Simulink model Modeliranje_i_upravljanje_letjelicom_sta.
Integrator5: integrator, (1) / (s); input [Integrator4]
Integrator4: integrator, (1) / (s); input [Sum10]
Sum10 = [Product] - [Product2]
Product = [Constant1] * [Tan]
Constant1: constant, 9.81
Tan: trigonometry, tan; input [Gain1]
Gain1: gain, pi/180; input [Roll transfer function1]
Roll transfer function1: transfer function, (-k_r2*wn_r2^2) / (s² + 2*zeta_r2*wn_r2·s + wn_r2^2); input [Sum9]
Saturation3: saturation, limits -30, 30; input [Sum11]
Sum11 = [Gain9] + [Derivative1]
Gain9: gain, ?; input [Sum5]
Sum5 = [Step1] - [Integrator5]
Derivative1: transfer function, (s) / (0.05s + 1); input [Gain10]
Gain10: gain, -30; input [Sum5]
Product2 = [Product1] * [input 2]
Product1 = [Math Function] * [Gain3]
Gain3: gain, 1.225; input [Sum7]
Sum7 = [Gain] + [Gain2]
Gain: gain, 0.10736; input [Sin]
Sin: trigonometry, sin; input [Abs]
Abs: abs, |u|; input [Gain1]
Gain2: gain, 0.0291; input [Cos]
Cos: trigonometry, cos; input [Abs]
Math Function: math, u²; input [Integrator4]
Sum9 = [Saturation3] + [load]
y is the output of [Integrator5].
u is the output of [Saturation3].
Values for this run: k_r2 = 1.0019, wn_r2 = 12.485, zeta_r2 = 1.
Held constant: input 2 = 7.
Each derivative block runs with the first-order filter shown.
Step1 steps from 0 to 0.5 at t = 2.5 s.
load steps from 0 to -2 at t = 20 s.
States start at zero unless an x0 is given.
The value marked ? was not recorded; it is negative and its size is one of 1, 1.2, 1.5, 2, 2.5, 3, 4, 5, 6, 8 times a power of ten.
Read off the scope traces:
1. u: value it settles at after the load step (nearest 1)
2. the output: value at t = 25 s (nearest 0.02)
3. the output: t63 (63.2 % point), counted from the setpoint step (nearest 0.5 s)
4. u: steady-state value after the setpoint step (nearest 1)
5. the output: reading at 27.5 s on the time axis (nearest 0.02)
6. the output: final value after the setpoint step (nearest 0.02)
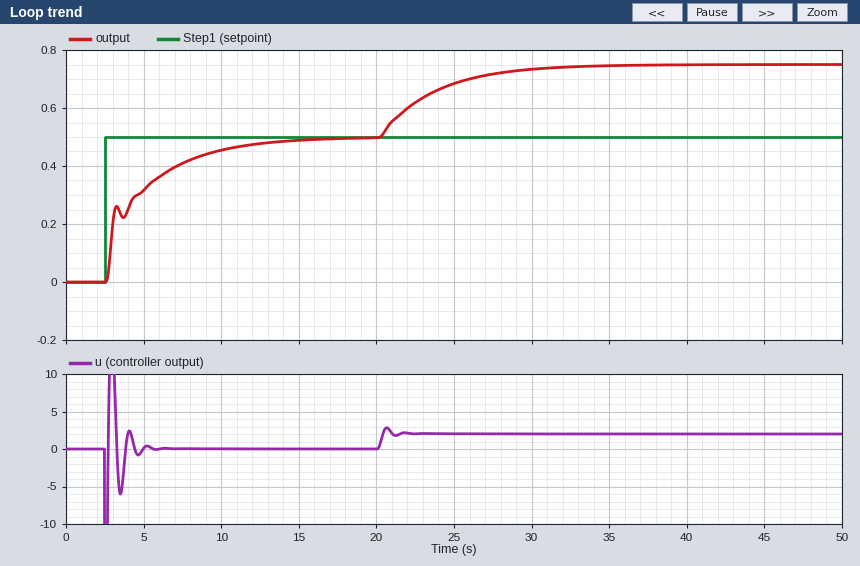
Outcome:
2
0.68
2.5 s
0
0.72
0.50
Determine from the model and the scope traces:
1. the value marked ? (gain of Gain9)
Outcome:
-8
